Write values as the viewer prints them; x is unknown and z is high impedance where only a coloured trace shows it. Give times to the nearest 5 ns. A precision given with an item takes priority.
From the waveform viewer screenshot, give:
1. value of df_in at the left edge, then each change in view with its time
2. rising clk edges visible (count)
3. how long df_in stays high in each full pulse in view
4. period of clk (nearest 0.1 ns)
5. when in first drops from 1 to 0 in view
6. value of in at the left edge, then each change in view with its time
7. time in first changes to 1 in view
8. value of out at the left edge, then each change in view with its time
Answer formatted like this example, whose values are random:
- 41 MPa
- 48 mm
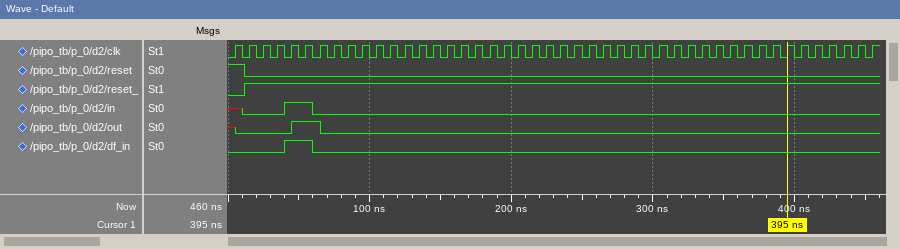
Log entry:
- 0, 1 at 40 ns, 0 at 60 ns
- 46
- 20 ns
- 10 ns
- 60 ns
- x, 0 at 10 ns, 1 at 40 ns, 0 at 60 ns
- 40 ns
- x, 0 at 5 ns, 1 at 45 ns, 0 at 65 ns
